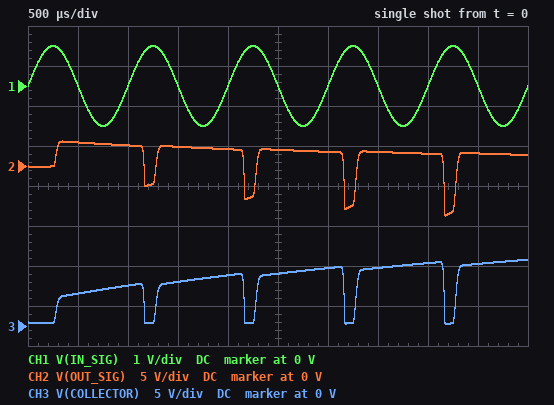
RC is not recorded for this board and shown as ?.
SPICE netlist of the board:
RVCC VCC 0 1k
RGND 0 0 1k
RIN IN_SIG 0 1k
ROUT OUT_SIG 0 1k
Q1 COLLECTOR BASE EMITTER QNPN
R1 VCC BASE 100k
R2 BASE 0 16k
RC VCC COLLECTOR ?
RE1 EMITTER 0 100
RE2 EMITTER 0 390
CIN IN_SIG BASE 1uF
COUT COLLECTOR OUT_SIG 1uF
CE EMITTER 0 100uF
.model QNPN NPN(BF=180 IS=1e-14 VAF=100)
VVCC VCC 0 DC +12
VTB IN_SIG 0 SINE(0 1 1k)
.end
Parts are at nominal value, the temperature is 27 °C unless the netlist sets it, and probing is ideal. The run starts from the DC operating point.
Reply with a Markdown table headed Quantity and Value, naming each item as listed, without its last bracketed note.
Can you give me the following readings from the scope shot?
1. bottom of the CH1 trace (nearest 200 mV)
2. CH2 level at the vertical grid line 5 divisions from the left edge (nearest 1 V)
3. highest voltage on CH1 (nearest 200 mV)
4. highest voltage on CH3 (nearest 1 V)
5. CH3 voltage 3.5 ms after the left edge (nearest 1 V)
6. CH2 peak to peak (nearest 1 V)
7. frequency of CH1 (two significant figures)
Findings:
| Quantity | Value |
|---|---|
| bottom of the CH1 trace | -1.0 V |
| CH2 level at the vertical grid line 5 divisions from the left edge | 2 V |
| highest voltage on CH1 | 1.0 V |
| highest voltage on CH3 | 8 V |
| CH3 voltage 3.5 ms after the left edge | 7 V |
| CH2 peak to peak | 9 V |
| frequency of CH1 | 1.0 kHz |
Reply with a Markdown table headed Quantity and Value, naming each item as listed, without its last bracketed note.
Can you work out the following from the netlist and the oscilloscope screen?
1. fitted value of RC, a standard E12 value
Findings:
| Quantity | Value |
|---|---|
| fitted value of RC, a standard E12 value | 2.7 kΩ |
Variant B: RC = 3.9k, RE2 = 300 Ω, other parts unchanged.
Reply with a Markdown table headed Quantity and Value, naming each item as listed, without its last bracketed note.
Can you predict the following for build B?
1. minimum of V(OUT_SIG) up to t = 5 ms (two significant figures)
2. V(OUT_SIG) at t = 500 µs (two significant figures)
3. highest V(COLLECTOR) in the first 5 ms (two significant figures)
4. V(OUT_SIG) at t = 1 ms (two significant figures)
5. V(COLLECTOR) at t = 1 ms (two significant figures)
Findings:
| Quantity | Value |
|---|---|
| minimum of V(OUT_SIG) up to t = 5 ms | -5.2 V |
| V(OUT_SIG) at t = 500 µs | 2.3 V |
| highest V(COLLECTOR) in the first 5 ms | 7.1 V |
| V(OUT_SIG) at t = 1 ms | 2.1 V |
| V(COLLECTOR) at t = 1 ms | 4.0 V |
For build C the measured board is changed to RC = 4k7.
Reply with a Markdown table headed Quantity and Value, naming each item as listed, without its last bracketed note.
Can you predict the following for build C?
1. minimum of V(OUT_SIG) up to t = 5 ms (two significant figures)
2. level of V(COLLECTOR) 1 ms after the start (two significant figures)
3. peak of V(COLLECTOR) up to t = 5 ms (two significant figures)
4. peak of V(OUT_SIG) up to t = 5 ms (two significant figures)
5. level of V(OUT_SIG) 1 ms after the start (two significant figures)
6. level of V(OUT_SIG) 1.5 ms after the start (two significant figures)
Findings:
| Quantity | Value |
|---|---|
| minimum of V(OUT_SIG) up to t = 5 ms | -4.6 V |
| level of V(COLLECTOR) 1 ms after the start | 3.5 V |
| peak of V(COLLECTOR) up to t = 5 ms | 6.4 V |
| peak of V(OUT_SIG) up to t = 5 ms | 2.0 V |
| level of V(OUT_SIG) 1 ms after the start | 1.8 V |
| level of V(OUT_SIG) 1.5 ms after the start | 1.7 V |
